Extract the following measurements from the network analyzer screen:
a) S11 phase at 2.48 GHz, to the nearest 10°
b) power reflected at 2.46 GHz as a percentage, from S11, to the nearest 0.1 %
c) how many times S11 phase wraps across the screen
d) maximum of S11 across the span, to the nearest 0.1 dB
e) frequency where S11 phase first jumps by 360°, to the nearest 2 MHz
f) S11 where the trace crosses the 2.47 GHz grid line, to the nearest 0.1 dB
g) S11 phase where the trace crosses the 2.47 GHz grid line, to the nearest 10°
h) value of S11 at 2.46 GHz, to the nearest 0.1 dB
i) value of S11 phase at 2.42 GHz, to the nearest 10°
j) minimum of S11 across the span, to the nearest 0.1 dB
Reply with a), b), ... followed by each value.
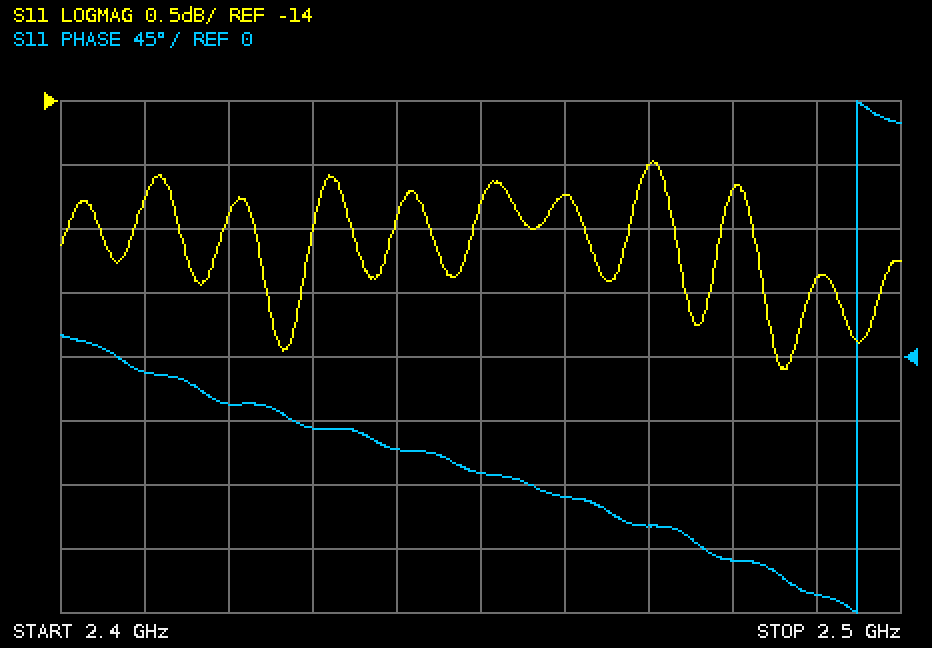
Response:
a) -140°
b) 3.4 %
c) 1
d) -14.5 dB
e) 2.494 GHz
f) -14.5 dB
g) -120°
h) -14.7 dB
i) -30°
j) -16.1 dB
